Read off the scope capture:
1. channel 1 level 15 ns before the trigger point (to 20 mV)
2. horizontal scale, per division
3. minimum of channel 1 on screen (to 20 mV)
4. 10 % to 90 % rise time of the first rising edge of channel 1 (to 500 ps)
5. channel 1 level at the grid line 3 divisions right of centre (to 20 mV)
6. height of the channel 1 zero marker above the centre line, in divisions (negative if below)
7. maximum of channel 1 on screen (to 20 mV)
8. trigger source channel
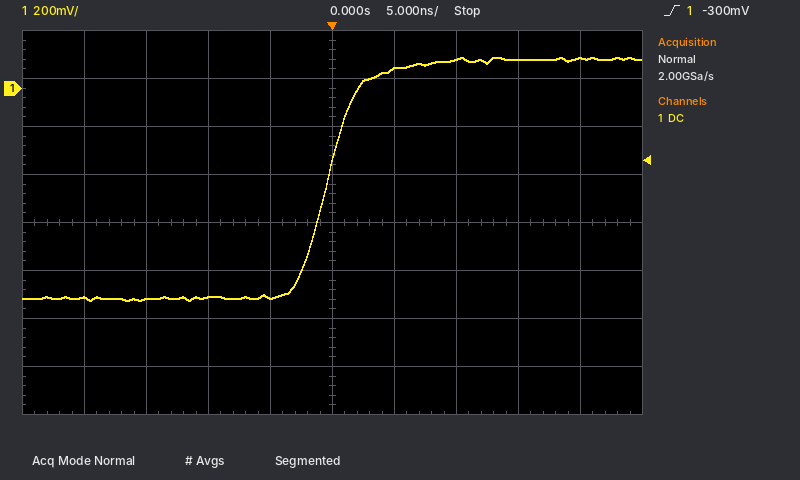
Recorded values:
-880 mV
5 ns
-880 mV
5.0 ns
120 mV
+2.8 div
120 mV
channel 1
